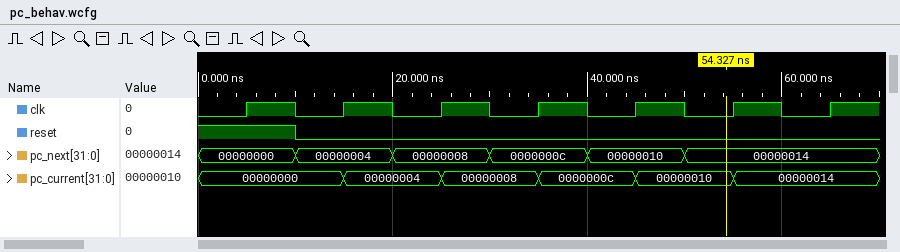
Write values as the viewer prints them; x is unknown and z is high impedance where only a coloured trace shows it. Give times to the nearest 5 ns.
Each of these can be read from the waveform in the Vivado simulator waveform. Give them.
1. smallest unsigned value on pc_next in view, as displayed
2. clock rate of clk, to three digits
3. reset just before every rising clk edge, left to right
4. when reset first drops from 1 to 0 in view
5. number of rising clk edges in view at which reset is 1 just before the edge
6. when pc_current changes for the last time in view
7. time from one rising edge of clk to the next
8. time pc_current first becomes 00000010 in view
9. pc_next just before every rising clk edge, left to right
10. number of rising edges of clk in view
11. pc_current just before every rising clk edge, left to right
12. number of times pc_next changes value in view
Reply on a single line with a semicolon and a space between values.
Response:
00000000; 100 MHz; 1 0 0 0 0 0 0; 10 ns; 1; 55 ns; 10 ns; 45 ns; 00000000, 00000004, 00000008, 0000000c, 00000010, 00000014, 00000014; 7; 00000000, 00000000, 00000004, 00000008, 0000000c, 00000010, 00000014; 5
